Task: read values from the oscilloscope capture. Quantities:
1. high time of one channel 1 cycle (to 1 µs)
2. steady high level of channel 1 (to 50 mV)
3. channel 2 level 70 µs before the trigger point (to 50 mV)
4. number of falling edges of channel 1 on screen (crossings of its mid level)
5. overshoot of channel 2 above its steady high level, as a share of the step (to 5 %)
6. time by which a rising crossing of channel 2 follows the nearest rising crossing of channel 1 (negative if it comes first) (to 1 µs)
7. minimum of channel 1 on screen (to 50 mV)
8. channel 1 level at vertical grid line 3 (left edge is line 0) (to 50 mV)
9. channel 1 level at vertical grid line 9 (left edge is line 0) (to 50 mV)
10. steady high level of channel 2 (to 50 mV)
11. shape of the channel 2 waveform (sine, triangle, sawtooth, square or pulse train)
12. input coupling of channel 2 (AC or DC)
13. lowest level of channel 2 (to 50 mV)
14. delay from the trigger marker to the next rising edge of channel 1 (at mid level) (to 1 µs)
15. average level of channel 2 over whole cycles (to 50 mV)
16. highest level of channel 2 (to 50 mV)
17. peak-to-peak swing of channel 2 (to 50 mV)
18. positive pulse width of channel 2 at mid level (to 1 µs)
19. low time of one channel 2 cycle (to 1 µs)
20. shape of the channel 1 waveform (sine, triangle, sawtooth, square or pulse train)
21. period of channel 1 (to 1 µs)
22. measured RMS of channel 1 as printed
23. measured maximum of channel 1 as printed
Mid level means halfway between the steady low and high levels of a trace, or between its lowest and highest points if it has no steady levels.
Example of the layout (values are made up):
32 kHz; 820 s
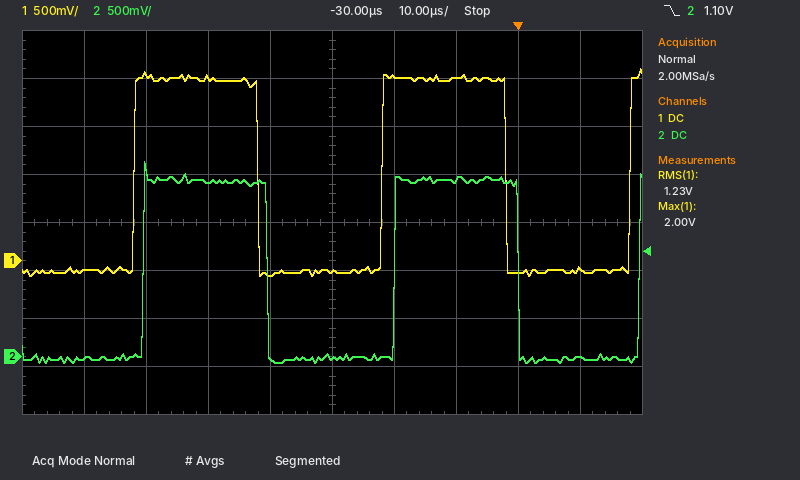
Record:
20 µs; 1.90 V; 0 mV; 2; 10 %; +2 µs; -150 mV; 1.90 V; -100 mV; 1.85 V; square; DC; -50 mV; 18 µs; 900 mV; 2.05 V; 2.10 V; 20 µs; 20 µs; square; 40 µs; 1.23 V; 2.00 V
